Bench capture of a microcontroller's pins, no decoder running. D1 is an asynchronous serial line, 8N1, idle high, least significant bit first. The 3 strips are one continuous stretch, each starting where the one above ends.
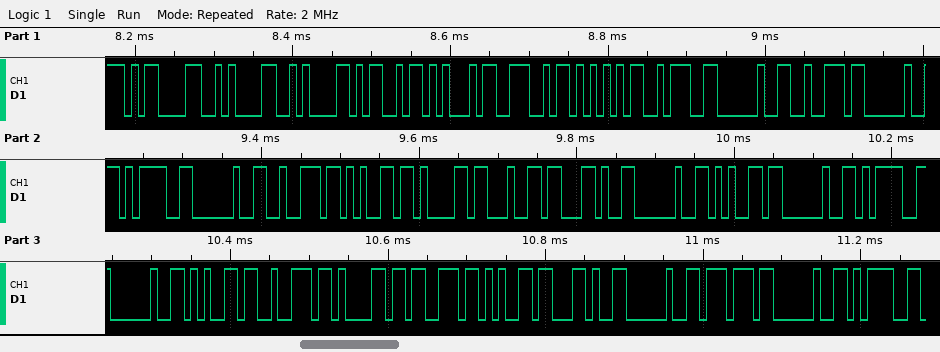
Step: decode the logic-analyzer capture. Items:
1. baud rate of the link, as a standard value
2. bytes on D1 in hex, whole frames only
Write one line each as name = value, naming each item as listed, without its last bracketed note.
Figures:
baud rate of the link, as a standard value = 115200 baud
bytes on D1 in hex, whole frames only = 0x0D 0x0A 0x0A 0x4D 0x45 0x4E 0x55 0x3A 0x20 0x72 0x20 0x3D 0x20 0x72 0x65 0x61 0x64 0x2C 0x20 0x65 0x20 0x3D 0x20 0x65 0x72 0x61 0x73 0x65 0x2C 0x20 0x77 0x20 0x3D
